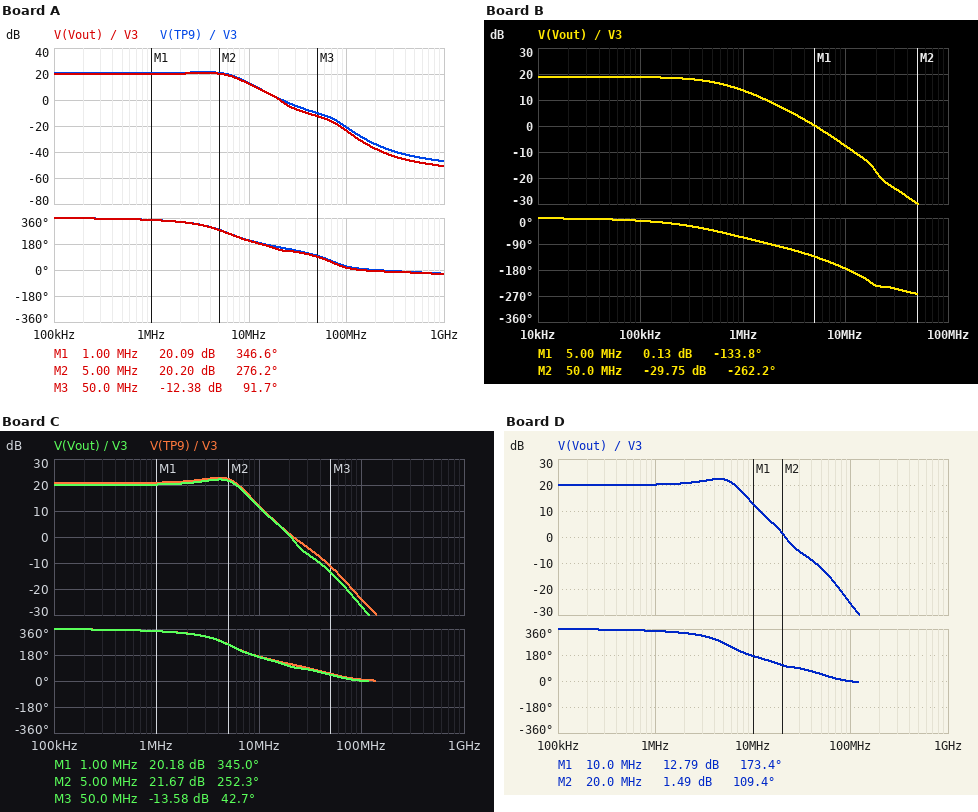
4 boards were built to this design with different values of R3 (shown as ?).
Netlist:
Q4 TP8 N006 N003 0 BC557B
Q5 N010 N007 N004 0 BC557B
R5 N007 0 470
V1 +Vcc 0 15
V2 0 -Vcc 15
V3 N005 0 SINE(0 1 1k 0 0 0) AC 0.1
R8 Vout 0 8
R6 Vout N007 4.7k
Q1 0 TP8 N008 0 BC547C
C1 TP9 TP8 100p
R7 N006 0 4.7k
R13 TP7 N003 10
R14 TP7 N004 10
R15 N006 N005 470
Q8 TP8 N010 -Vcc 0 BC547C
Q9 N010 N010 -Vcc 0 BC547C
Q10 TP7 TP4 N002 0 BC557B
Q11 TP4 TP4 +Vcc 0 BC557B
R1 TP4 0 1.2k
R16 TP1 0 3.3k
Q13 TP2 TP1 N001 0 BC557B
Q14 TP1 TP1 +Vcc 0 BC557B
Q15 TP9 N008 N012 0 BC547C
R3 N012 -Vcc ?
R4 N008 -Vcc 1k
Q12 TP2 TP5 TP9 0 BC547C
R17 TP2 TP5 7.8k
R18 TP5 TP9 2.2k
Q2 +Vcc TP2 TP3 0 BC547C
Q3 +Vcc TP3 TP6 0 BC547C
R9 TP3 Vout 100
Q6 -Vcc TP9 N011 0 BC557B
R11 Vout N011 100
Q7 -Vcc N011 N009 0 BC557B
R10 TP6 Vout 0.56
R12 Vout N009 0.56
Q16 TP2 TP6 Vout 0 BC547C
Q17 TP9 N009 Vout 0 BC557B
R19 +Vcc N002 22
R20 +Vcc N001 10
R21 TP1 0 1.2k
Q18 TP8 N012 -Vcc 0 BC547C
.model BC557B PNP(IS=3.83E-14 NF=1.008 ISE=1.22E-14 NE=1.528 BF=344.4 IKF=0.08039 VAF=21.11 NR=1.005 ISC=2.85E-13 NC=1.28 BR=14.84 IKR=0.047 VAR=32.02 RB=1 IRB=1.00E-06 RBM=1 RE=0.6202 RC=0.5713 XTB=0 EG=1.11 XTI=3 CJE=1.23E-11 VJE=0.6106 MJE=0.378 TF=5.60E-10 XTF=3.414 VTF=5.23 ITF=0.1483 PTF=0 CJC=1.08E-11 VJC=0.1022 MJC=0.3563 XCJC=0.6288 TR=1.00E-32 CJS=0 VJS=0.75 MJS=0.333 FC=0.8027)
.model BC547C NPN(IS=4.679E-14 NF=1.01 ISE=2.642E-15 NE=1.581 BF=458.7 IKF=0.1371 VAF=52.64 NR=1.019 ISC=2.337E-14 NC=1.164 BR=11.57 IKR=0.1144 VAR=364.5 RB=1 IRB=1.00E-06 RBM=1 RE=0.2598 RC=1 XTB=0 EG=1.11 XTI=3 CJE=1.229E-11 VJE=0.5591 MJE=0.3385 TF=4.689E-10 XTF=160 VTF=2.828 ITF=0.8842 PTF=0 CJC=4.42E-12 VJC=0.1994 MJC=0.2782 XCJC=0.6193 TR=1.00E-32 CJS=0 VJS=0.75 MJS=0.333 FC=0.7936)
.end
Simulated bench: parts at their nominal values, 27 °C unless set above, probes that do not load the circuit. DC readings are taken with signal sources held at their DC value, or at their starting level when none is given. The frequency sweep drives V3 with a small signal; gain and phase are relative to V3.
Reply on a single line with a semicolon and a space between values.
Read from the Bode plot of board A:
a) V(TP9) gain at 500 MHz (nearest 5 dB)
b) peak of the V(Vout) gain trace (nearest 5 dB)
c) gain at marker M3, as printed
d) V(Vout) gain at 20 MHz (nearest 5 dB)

-45 dB; 20 dB; -12.38 dB; 0 dB
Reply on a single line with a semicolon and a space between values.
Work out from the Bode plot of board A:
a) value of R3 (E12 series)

33 Ω
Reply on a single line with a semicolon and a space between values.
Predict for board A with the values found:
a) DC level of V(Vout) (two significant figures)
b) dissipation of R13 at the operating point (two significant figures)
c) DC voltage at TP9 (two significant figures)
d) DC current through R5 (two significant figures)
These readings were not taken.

13 mV; 19 µW; -1.6 V; 4.7 µA
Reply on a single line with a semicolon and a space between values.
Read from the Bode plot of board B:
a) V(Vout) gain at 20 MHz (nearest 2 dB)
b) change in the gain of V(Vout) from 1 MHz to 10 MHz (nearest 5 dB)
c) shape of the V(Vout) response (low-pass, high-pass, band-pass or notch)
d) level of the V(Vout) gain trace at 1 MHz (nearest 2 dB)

-18 dB; -20 dB; low-pass; 14 dB
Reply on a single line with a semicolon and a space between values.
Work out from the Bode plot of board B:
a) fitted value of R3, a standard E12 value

120 Ω
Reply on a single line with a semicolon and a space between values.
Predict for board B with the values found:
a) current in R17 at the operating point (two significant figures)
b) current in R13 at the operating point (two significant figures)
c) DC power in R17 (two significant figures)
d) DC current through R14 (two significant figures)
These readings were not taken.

310 µA; 2.0 mA; 760 µW; 730 µA
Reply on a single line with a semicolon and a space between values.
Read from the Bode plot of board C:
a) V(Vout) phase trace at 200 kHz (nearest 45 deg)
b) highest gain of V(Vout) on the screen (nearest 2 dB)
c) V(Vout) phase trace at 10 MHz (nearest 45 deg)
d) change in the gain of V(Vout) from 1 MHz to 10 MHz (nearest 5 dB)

360 deg; 22 dB; 180 deg; -10 dB
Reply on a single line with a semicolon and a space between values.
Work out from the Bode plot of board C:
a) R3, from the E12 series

100 Ω
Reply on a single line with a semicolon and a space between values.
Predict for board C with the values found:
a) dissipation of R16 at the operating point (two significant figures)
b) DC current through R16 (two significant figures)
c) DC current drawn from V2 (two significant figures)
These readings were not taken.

62 mW; 4.3 mA; 140 mA
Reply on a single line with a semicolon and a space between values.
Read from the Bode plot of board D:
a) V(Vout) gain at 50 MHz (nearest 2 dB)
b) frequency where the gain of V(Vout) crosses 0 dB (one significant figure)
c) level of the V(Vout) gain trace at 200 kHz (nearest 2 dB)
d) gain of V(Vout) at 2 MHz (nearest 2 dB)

-12 dB; 20 MHz; 20 dB; 20 dB
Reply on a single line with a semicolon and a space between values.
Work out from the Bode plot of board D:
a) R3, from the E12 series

82 Ω
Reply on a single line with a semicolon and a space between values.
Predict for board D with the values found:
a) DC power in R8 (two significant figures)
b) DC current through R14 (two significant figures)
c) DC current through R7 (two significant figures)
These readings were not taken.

39 µW; 1.4 mA; 240 nA
